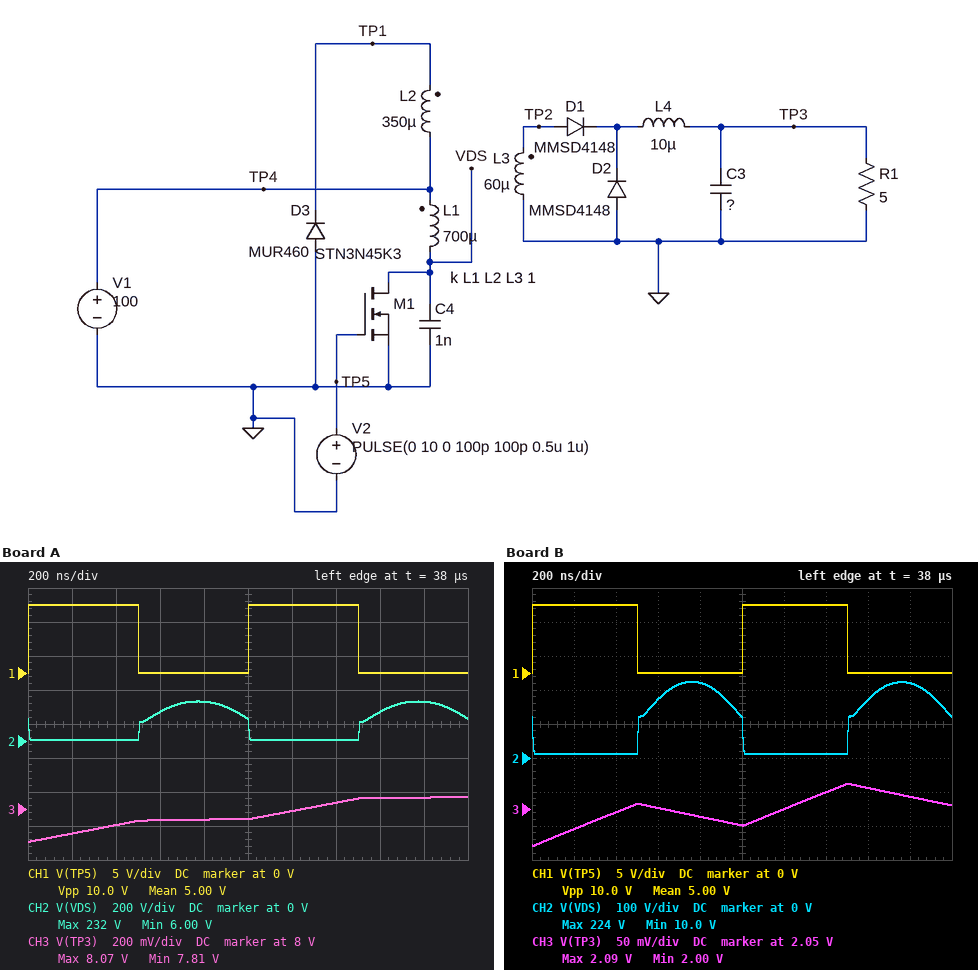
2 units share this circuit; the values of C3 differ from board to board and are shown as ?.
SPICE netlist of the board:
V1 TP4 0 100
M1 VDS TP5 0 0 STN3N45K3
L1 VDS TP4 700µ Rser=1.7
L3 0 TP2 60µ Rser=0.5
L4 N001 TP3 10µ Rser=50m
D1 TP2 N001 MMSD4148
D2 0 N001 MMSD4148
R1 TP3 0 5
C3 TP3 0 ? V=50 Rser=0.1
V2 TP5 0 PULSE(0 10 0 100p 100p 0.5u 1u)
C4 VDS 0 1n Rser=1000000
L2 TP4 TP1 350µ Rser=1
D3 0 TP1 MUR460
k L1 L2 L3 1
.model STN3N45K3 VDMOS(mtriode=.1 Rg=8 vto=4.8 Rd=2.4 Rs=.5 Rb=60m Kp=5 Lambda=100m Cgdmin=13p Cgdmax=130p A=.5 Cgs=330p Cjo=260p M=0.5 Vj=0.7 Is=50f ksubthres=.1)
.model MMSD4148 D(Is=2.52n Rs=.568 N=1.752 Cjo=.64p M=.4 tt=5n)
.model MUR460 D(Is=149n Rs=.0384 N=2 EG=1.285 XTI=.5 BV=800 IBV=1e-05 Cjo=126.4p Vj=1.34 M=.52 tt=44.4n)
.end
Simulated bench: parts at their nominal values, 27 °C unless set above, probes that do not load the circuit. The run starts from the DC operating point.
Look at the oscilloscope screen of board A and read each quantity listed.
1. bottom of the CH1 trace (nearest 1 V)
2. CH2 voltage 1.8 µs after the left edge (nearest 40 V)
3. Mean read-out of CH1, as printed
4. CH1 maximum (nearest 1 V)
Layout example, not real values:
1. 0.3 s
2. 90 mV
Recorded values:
1. 0 V
2. 240 V
3. 5.00 V
4. 10 V
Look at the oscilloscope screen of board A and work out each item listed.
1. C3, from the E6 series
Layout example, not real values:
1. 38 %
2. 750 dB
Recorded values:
1. 33 µF
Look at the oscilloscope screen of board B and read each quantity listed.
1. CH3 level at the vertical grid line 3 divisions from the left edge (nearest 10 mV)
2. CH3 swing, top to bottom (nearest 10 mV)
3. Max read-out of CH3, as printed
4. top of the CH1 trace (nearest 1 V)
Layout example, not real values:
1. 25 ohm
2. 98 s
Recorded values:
1. 2.05 V
2. 90 mV
3. 2.09 V
4. 10 V
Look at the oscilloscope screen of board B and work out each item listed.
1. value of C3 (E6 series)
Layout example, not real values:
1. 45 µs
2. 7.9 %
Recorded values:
1. 330 µF
